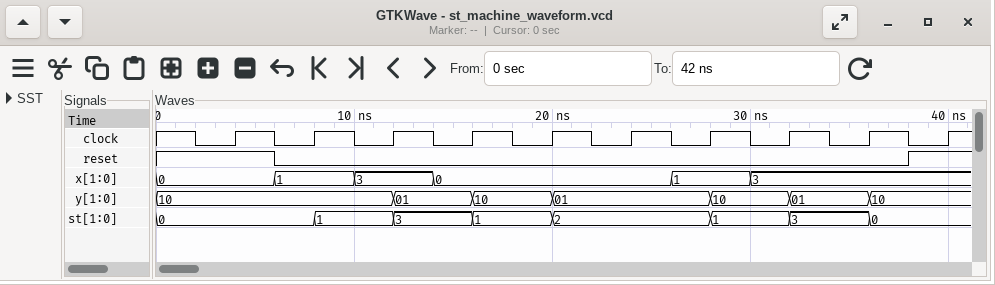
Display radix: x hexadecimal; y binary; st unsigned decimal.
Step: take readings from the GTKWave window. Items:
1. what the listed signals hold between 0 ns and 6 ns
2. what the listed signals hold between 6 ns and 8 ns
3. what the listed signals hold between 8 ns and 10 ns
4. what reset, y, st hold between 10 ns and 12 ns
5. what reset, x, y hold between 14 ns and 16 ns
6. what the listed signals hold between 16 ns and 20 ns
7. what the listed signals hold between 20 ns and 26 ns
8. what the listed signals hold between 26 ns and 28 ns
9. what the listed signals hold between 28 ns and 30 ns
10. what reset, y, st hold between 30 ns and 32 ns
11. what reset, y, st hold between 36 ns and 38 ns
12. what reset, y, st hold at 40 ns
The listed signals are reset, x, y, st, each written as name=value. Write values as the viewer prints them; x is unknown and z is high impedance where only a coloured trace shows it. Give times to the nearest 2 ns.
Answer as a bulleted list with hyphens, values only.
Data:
- reset=1, x=0, y=10, st=0
- reset=0, x=1, y=10, st=0
- reset=0, x=1, y=10, st=1
- reset=0, y=10, st=1
- reset=0, x=0, y=01
- reset=0, x=0, y=10, st=1
- reset=0, x=0, y=01, st=2
- reset=0, x=1, y=01, st=2
- reset=0, x=1, y=10, st=1
- reset=0, y=10, st=1
- reset=0, y=10, st=0
- reset=1, y=10, st=0
